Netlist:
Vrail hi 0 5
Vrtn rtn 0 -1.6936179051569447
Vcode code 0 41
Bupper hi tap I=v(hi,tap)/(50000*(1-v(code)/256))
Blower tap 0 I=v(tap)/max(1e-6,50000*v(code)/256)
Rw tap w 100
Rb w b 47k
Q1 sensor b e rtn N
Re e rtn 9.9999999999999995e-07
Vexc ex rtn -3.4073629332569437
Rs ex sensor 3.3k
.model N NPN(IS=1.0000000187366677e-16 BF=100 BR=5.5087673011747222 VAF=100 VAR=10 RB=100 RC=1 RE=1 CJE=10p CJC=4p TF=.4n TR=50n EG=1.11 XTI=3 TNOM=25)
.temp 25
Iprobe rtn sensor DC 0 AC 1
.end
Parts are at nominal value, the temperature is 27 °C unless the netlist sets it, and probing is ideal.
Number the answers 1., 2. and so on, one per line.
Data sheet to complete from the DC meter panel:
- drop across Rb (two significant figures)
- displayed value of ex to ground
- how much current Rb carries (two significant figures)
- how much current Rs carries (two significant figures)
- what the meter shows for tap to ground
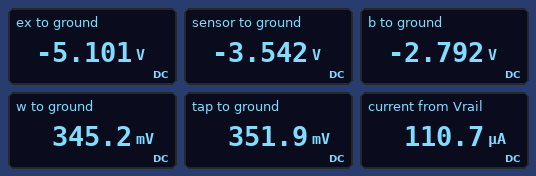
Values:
1. 3.1 V
2. -5.101 V
3. 67 µA
4. 470 µA
5. 351.9 mV
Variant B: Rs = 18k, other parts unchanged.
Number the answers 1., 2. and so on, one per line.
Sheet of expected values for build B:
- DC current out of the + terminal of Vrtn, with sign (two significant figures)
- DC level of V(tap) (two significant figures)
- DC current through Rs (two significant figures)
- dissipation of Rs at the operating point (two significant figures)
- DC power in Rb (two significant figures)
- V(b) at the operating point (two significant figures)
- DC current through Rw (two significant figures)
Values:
1. -34 µA
2. 570 mV
3. 190 µA
4. 620 µW
5. 54 µW
6. -1.0 V
7. 34 µA
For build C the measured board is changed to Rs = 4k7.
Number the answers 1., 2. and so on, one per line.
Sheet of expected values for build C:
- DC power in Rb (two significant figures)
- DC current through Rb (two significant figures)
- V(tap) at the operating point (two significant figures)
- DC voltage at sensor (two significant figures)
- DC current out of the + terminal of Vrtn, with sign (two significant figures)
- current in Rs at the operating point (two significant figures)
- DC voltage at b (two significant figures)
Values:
1. 170 µW
2. 60 µA
3. 400 mV
4. -3.2 V
5. -60 µA
6. 410 µA
7. -2.4 V
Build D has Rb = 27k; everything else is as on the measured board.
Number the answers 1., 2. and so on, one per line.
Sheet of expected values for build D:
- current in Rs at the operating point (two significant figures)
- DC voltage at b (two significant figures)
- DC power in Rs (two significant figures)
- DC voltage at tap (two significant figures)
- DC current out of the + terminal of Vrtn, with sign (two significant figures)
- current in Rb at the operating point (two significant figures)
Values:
1. 620 µA
2. -2.3 V
3. 1.3 mW
4. 190 mV
5. -91 µA
6. 91 µA
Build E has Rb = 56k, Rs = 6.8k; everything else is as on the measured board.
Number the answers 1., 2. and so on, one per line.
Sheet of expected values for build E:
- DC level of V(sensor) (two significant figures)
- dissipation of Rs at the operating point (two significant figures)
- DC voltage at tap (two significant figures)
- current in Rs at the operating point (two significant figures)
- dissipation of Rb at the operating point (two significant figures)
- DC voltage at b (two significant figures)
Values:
1. -2.9 V
2. 700 µW
3. 480 mV
4. 320 µA
5. 130 µW
6. -2.2 V
